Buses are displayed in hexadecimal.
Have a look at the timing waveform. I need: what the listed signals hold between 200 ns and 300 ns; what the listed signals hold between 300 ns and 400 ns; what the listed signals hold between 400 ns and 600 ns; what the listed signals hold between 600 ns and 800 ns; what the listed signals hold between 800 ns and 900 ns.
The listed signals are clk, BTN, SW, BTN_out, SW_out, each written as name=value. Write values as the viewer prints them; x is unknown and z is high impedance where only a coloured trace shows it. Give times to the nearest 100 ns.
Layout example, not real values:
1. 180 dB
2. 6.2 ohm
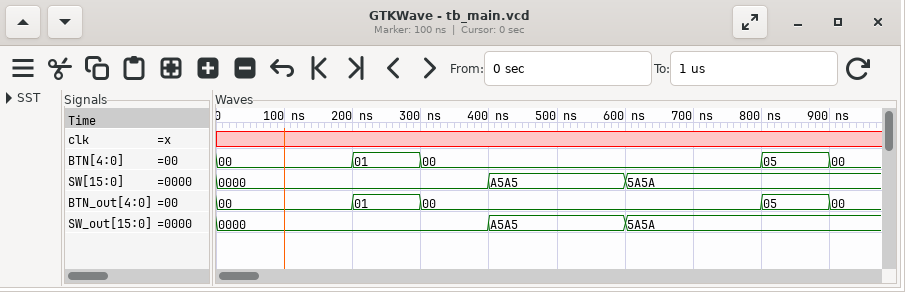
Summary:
1. clk=x, BTN=01, SW=0000, BTN_out=01, SW_out=0000
2. clk=x, BTN=00, SW=0000, BTN_out=00, SW_out=0000
3. clk=x, BTN=00, SW=A5A5, BTN_out=00, SW_out=A5A5
4. clk=x, BTN=00, SW=5A5A, BTN_out=00, SW_out=5A5A
5. clk=x, BTN=05, SW=5A5A, BTN_out=05, SW_out=5A5A
